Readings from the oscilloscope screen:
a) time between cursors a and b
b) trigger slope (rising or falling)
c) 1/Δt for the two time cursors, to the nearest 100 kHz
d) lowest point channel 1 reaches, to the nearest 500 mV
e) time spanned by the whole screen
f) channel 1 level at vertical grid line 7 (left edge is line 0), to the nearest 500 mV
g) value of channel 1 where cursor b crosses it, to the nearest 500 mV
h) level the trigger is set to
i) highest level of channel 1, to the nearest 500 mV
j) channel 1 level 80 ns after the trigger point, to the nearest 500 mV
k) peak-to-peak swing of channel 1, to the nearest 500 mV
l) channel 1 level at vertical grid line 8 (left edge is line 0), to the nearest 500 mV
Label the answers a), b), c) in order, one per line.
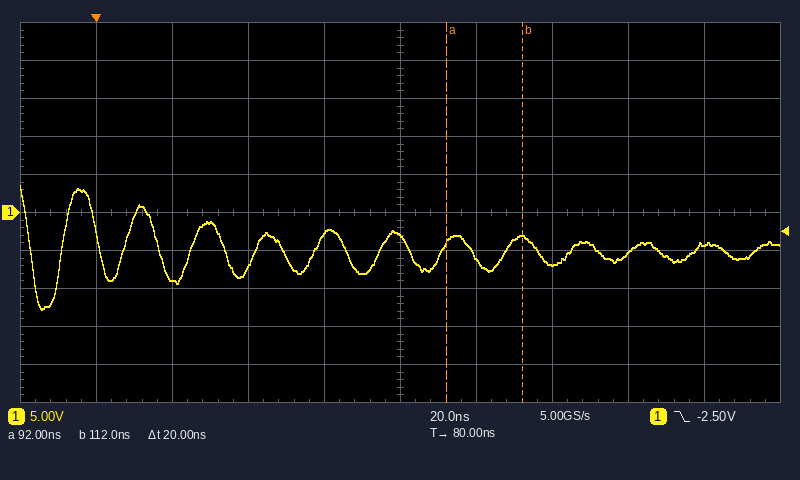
a) 20 ns
b) falling
c) 50.0 MHz
d) -13.0 V
e) 200 ns
f) -7.0 V
g) -3.0 V
h) -2.50 V
i) 3.5 V
j) -3.0 V
k) 16.5 V
l) -5.5 V
